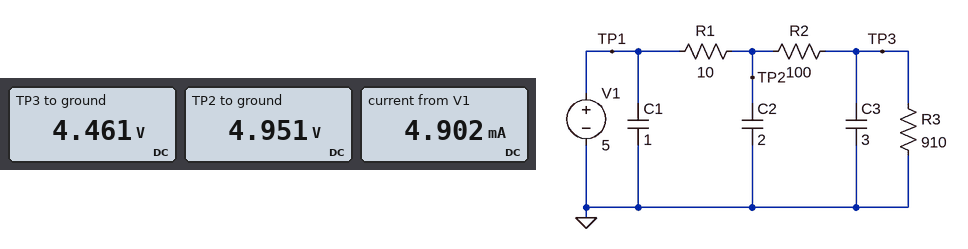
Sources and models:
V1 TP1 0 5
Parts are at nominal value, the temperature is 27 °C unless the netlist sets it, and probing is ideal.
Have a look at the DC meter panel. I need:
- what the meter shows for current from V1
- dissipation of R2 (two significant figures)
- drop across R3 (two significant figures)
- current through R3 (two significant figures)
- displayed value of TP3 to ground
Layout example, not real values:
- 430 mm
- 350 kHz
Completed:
- 4.902 mA
- 2.4 mW
- 4.5 V
- 4.9 mA
- 4.461 V
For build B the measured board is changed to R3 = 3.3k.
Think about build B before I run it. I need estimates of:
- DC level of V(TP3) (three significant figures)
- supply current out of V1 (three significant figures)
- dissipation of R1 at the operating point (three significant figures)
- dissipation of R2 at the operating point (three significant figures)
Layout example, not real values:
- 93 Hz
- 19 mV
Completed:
- 4.84 V
- 1.47 mA
- 21.5 µW
- 215 µW
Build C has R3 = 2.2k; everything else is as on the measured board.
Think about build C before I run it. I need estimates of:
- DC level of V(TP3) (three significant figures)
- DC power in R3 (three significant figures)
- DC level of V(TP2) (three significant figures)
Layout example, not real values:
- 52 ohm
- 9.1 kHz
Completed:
- 4.76 V
- 10.3 mW
- 4.98 V
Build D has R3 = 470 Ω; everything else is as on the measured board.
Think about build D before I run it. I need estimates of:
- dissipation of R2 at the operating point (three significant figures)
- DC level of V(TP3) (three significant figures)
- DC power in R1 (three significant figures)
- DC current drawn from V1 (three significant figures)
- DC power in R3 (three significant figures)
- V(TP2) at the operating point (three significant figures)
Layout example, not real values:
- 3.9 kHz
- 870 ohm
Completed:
- 7.43 mW
- 4.05 V
- 743 µW
- 8.62 mA
- 34.9 mW
- 4.91 V
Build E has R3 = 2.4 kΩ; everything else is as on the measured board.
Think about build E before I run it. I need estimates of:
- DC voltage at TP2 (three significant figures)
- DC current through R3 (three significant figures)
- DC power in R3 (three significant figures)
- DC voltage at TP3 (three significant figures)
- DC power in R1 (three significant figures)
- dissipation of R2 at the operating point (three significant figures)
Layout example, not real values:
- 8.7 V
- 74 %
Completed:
- 4.98 V
- 1.99 mA
- 9.52 mW
- 4.78 V
- 39.7 µW
- 397 µW
